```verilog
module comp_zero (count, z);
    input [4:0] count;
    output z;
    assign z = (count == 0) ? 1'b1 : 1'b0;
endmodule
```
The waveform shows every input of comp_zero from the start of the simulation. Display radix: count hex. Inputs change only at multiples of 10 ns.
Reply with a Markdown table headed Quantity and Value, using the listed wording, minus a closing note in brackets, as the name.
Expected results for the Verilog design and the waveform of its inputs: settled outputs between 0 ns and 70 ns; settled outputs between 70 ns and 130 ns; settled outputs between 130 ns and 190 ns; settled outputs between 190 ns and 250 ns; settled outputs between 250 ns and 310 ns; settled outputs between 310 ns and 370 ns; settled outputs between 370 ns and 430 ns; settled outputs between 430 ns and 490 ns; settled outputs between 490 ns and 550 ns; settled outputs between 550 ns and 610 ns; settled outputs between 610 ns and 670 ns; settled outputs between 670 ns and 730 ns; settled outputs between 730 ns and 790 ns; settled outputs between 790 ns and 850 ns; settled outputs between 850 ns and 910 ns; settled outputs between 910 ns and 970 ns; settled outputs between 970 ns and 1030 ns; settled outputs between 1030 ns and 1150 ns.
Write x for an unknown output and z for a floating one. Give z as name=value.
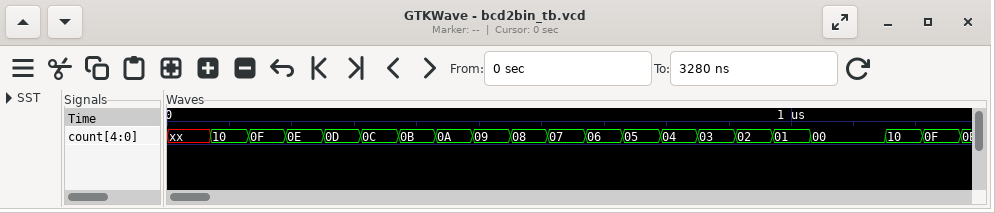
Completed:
| Quantity | Value |
|---|---|
| settled outputs between 0 ns and 70 ns | z=x |
| settled outputs between 70 ns and 130 ns | z=0 |
| settled outputs between 130 ns and 190 ns | z=0 |
| settled outputs between 190 ns and 250 ns | z=0 |
| settled outputs between 250 ns and 310 ns | z=0 |
| settled outputs between 310 ns and 370 ns | z=0 |
| settled outputs between 370 ns and 430 ns | z=0 |
| settled outputs between 430 ns and 490 ns | z=0 |
| settled outputs between 490 ns and 550 ns | z=0 |
| settled outputs between 550 ns and 610 ns | z=0 |
| settled outputs between 610 ns and 670 ns | z=0 |
| settled outputs between 670 ns and 730 ns | z=0 |
| settled outputs between 730 ns and 790 ns | z=0 |
| settled outputs between 790 ns and 850 ns | z=0 |
| settled outputs between 850 ns and 910 ns | z=0 |
| settled outputs between 910 ns and 970 ns | z=0 |
| settled outputs between 970 ns and 1030 ns | z=0 |
| settled outputs between 1030 ns and 1150 ns | z=1 |
